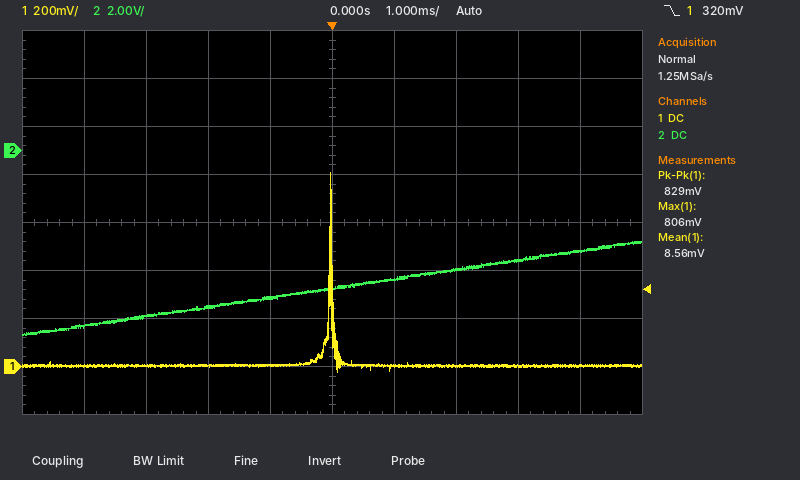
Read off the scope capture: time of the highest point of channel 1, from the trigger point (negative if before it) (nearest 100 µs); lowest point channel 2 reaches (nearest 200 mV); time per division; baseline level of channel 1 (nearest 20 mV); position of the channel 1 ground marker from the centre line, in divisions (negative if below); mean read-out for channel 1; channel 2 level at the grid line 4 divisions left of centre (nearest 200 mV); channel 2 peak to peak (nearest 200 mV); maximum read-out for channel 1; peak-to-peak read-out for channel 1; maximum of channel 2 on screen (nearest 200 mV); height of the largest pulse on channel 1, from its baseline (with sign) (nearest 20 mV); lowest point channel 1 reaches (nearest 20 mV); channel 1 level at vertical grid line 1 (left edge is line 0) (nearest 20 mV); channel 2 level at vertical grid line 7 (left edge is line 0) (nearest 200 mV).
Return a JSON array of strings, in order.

["0.0 ms", "-7.8 V", "1 ms", "0 mV", "-3.0 div", "8.56 mV", "-7.4 V", "4.0 V", "806 mV", "829 mV", "-3.8 V", "+800 mV", "-20 mV", "0 mV", "-5.0 V"]
